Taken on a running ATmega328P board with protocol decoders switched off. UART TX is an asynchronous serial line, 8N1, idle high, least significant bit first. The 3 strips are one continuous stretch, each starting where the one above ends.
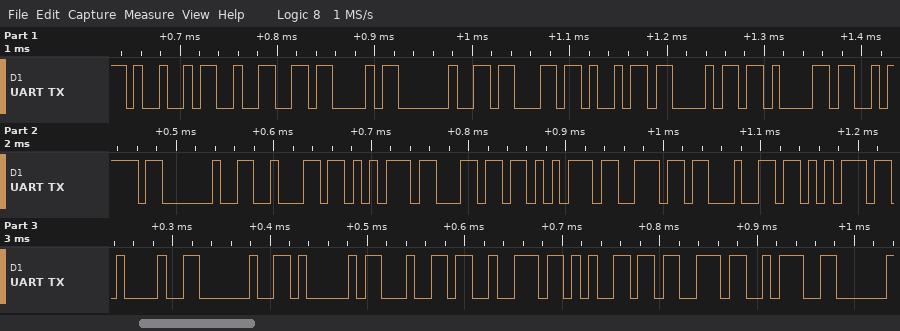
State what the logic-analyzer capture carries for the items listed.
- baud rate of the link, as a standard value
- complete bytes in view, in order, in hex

115200 baud
49 32 43 20 63 69 68 61 7A 20 62 75 6C 75 6E 64 75 21 20 41 64 72 65 73 3A
